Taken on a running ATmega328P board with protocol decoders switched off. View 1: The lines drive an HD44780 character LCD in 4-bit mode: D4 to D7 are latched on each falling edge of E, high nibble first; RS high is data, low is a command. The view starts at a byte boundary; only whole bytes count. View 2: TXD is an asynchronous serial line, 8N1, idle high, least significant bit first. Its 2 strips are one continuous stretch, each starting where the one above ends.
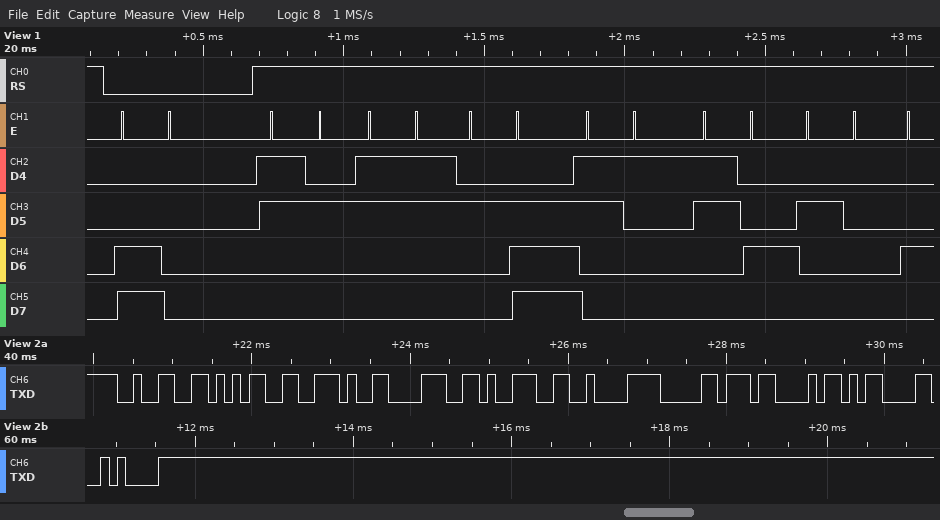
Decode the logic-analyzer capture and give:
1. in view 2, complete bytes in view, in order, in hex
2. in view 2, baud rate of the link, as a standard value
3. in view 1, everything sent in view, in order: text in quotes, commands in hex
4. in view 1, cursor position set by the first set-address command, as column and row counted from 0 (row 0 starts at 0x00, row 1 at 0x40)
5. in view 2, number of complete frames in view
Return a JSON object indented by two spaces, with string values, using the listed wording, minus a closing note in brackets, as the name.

{
  "in view 2, complete bytes in view, in order, in hex": "32 35 2E 38 39 C2 B0 43 0D 0A",
  "in view 2, baud rate of the link, as a standard value": "9600 baud",
  "in view 1, everything sent in view, in order: text in quotes, commands in hex": "0xC0 \"23.14 \"",
  "in view 1, cursor position set by the first set-address command, as column and row counted from 0": "column 0, row 1",
  "in view 2, number of complete frames in view": "10"
}
